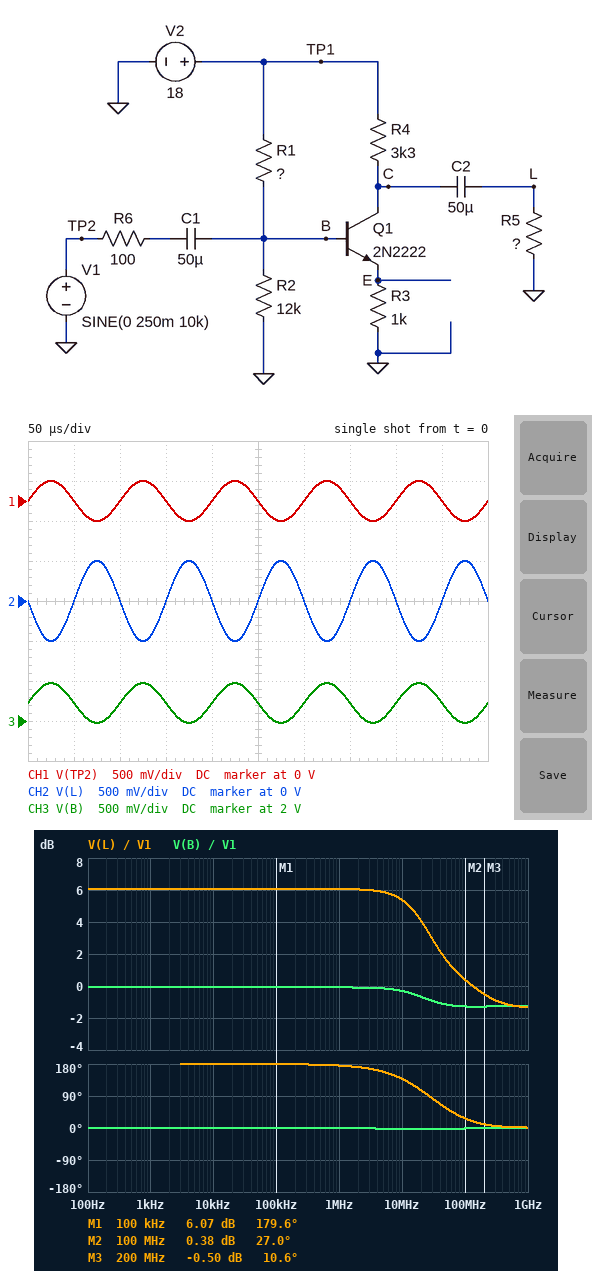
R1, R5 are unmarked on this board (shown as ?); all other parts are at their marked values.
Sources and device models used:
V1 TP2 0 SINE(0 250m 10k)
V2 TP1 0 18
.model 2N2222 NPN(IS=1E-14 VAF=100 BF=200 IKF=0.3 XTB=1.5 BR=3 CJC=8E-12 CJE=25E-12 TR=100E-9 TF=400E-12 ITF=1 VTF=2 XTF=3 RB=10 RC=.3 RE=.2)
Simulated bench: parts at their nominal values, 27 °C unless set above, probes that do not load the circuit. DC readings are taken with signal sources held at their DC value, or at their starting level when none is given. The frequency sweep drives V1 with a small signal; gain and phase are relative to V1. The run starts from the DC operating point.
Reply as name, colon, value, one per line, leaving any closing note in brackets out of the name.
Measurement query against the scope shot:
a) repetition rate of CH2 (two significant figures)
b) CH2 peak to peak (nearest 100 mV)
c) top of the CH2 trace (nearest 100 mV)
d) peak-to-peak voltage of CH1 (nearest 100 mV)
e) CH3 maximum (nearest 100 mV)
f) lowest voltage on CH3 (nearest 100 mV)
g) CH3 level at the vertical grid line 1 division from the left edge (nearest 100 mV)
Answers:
repetition rate of CH2: 10 kHz
CH2 peak to peak: 1.0 V
top of the CH2 trace: 500 mV
peak-to-peak voltage of CH1: 500 mV
CH3 maximum: 2.5 V
lowest voltage on CH3: 2.0 V
CH3 level at the vertical grid line 1 division from the left edge: 2.2 V
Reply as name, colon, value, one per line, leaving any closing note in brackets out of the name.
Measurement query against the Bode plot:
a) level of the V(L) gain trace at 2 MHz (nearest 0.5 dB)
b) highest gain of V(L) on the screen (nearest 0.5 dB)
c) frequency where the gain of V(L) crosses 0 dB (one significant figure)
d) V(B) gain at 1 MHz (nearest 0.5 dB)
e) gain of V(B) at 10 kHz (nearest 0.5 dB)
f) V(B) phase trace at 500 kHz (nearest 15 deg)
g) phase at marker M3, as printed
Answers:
level of the V(L) gain trace at 2 MHz: 6.0 dB
highest gain of V(L) on the screen: 6.0 dB
frequency where the gain of V(L) crosses 0 dB: 100 MHz
V(B) gain at 1 MHz: 0 dB
gain of V(B) at 10 kHz: 0 dB
V(B) phase trace at 500 kHz: 0 deg
phase at marker M3, as printed: 10.6 deg
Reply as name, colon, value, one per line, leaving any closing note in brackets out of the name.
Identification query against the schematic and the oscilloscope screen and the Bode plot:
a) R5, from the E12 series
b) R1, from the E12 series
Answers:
R5, from the E12 series: 5.6 kΩ
R1, from the E12 series: 82 kΩ
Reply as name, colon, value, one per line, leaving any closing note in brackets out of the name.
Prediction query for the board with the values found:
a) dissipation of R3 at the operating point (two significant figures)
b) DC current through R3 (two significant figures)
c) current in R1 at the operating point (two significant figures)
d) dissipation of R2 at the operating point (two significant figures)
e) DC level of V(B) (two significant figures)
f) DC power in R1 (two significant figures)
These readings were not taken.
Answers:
dissipation of R3 at the operating point: 2.4 mW
DC current through R3: 1.6 mA
current in R1 at the operating point: 190 µA
dissipation of R2 at the operating point: 410 µW
DC level of V(B): 2.2 V
DC power in R1: 3.0 mW
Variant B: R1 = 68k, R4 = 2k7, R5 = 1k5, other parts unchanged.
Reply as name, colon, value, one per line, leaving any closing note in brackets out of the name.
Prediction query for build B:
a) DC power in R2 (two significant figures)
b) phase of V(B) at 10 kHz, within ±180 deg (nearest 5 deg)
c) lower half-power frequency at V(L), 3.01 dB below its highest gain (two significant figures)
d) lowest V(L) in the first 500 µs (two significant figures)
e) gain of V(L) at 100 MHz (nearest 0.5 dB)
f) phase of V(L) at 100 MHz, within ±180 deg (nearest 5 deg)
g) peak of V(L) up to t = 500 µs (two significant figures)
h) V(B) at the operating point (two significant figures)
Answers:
DC power in R2: 570 µW
phase of V(B) at 10 kHz, within ±180 deg: 0 deg
lower half-power frequency at V(L), 3.01 dB below its highest gain: 880 mHz
lowest V(L) in the first 500 µs: -230 mV
gain of V(L) at 100 MHz: -0.5 dB
phase of V(L) at 100 MHz, within ±180 deg: 40 deg
peak of V(L) up to t = 500 µs: 230 mV
V(B) at the operating point: 2.6 V
